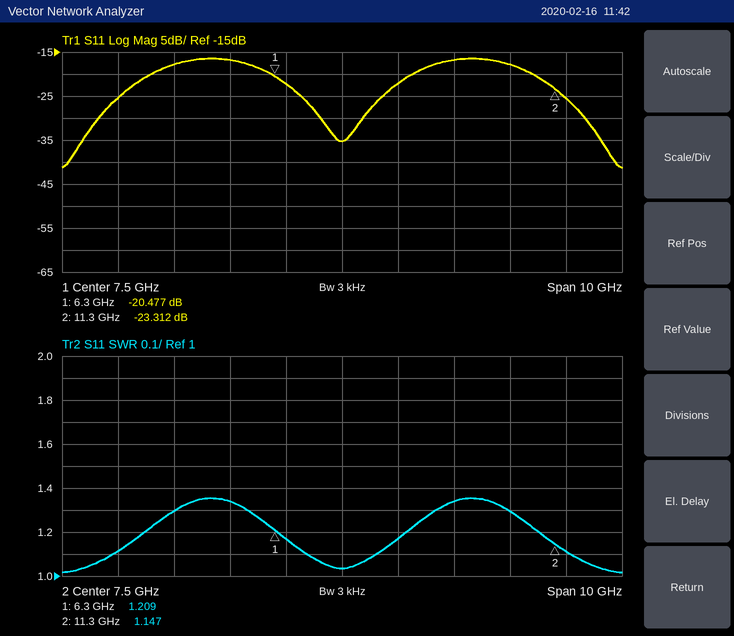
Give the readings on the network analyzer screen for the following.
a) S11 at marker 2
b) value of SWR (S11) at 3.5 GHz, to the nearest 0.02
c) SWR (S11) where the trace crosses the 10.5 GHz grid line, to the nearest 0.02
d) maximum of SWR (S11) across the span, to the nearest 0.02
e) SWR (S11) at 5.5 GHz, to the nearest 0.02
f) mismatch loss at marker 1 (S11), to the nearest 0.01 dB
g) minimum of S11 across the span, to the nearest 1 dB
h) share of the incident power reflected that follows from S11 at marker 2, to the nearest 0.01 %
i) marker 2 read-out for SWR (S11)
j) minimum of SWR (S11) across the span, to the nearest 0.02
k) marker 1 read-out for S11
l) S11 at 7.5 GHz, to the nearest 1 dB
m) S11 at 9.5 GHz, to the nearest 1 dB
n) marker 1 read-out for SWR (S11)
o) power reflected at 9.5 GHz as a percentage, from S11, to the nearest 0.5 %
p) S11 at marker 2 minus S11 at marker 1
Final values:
-23.312 dB
1.12
1.30
1.36
1.34
0.04 dB
-41 dB
0.47 %
1.147
1.02
-20.477 dB
-35 dB
-17 dB
1.209
2.0 %
-2.835 dB
